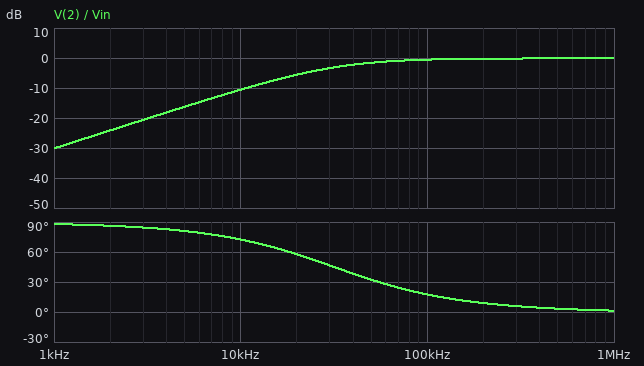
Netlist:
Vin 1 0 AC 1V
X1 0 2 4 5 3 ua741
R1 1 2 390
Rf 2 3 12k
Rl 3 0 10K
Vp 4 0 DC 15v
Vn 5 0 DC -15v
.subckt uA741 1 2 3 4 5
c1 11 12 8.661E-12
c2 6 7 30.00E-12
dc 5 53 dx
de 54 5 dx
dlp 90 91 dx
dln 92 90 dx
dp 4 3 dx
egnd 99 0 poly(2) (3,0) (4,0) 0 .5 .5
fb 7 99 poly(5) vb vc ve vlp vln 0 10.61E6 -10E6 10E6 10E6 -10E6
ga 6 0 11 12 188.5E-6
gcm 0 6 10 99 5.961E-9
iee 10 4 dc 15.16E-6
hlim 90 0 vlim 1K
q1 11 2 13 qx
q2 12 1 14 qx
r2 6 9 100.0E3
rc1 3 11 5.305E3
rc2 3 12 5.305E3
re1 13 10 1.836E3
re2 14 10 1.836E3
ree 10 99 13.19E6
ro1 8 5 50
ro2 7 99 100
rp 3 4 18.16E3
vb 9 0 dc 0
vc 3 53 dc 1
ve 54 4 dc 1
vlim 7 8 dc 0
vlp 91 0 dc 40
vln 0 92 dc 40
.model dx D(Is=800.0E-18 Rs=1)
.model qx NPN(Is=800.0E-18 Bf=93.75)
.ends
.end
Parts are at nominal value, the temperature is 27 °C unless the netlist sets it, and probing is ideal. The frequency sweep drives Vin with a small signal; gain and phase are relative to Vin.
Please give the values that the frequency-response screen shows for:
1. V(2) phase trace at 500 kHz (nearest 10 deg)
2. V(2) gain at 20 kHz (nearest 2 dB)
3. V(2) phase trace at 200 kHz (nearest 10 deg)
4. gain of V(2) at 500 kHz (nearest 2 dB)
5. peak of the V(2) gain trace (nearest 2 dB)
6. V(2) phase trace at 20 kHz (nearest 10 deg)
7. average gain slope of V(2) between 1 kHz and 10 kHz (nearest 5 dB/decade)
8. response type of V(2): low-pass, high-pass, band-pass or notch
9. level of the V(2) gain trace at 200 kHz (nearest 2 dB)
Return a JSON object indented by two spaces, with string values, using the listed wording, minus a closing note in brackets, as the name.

{
  "V(2) phase trace at 500 kHz": "0 deg",
  "V(2) gain at 20 kHz": "-6 dB",
  "V(2) phase trace at 200 kHz": "10 deg",
  "gain of V(2) at 500 kHz": "0 dB",
  "peak of the V(2) gain trace": "0 dB",
  "V(2) phase trace at 20 kHz": "60 deg",
  "average gain slope of V(2) between 1 kHz and 10 kHz": "20 dB/decade",
  "response type of V(2): low-pass, high-pass, band-pass or notch": "high-pass",
  "level of the V(2) gain trace at 200 kHz": "0 dB"
}
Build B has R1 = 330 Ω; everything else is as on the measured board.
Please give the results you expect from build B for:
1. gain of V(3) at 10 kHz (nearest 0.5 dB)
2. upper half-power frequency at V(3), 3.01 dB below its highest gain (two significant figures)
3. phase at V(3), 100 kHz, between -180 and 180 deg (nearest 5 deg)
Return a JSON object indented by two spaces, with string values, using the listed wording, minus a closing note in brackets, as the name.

{
  "gain of V(3) at 10 kHz": "30.5 dB",
  "upper half-power frequency at V(3), 3.01 dB below its highest gain": "27 kHz",
  "phase at V(3), 100 kHz, between -180 and 180 deg": "100 deg"
}
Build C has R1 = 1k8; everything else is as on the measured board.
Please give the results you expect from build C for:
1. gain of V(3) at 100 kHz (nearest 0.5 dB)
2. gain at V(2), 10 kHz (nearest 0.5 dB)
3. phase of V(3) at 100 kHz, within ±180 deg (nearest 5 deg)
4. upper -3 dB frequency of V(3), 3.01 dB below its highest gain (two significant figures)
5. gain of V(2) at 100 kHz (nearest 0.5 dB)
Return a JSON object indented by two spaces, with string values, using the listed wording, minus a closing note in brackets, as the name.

{
  "gain of V(3) at 100 kHz": "14.5 dB",
  "gain at V(2), 10 kHz": "-23.5 dB",
  "phase of V(3) at 100 kHz, within ±180 deg": "140 deg",
  "upper -3 dB frequency of V(3), 3.01 dB below its highest gain": "140 kHz",
  "gain of V(2) at 100 kHz": "-5.0 dB"
}
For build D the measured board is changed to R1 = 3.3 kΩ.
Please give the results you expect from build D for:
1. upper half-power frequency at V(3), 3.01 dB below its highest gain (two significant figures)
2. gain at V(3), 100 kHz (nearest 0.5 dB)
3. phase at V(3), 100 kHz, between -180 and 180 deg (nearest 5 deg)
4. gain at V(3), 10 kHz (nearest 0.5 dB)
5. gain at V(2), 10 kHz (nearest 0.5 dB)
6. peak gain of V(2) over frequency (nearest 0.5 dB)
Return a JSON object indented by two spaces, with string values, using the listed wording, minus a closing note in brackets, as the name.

{
  "upper half-power frequency at V(3), 3.01 dB below its highest gain": "240 kHz",
  "gain at V(3), 100 kHz": "10.5 dB",
  "phase at V(3), 100 kHz, between -180 and 180 deg": "155 deg",
  "gain at V(3), 10 kHz": "11.0 dB",
  "gain at V(2), 10 kHz": "-28.5 dB",
  "peak gain of V(2) over frequency": "-1.5 dB"
}
